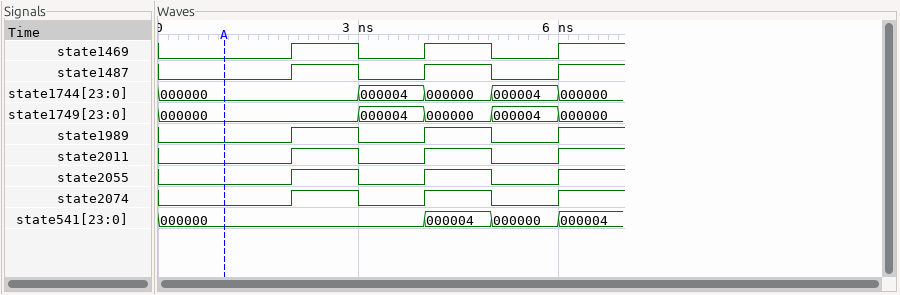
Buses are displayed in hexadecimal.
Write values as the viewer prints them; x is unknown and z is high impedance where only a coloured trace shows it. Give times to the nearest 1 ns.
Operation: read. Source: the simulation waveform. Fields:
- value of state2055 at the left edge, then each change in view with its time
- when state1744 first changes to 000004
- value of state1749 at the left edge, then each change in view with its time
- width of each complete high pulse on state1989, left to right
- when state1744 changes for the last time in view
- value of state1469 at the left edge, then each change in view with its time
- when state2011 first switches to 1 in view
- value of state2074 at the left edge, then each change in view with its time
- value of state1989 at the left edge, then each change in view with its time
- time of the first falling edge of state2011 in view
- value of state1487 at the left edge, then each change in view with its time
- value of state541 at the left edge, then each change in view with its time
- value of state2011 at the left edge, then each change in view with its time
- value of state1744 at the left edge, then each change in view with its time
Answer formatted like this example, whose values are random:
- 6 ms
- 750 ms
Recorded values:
- 0, 1 at 2 ns, 0 at 3 ns, 1 at 4 ns, 0 at 5 ns, 1 at 6 ns
- 3 ns
- 000000, 000004 at 3 ns, 000000 at 4 ns, 000004 at 5 ns, 000000 at 6 ns
- 1 ns, 1 ns
- 6 ns
- 0, 1 at 2 ns, 0 at 3 ns, 1 at 4 ns, 0 at 5 ns, 1 at 6 ns
- 2 ns
- 0, 1 at 2 ns, 0 at 3 ns, 1 at 4 ns, 0 at 5 ns, 1 at 6 ns
- 0, 1 at 2 ns, 0 at 3 ns, 1 at 4 ns, 0 at 5 ns, 1 at 6 ns
- 3 ns
- 0, 1 at 2 ns, 0 at 3 ns, 1 at 4 ns, 0 at 5 ns, 1 at 6 ns
- 000000, 000004 at 4 ns, 000000 at 5 ns, 000004 at 6 ns
- 0, 1 at 2 ns, 0 at 3 ns, 1 at 4 ns, 0 at 5 ns, 1 at 6 ns
- 000000, 000004 at 3 ns, 000000 at 4 ns, 000004 at 5 ns, 000000 at 6 ns
